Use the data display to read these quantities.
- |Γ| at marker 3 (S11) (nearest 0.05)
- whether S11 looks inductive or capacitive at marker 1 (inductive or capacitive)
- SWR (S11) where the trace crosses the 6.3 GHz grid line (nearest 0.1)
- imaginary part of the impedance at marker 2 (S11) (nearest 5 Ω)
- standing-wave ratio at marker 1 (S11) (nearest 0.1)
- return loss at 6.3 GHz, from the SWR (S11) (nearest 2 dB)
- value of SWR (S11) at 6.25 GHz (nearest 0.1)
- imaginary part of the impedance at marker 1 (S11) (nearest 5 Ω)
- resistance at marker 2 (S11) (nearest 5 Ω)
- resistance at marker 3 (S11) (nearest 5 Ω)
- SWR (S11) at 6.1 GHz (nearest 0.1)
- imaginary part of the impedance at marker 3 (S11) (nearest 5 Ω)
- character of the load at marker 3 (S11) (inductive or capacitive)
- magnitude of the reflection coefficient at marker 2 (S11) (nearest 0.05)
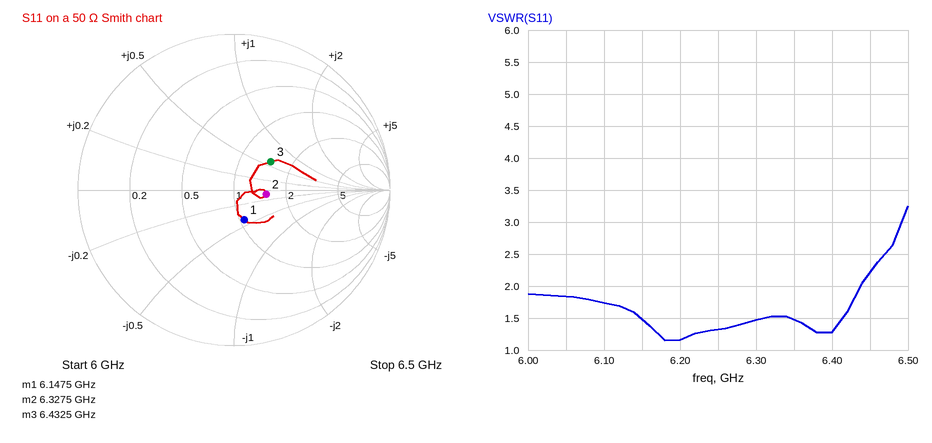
0.30
capacitive
1.5
-5 Ω
1.5
14 dB
1.3
-20 Ω
75 Ω
75 Ω
1.7
+30 Ω
inductive
0.20
